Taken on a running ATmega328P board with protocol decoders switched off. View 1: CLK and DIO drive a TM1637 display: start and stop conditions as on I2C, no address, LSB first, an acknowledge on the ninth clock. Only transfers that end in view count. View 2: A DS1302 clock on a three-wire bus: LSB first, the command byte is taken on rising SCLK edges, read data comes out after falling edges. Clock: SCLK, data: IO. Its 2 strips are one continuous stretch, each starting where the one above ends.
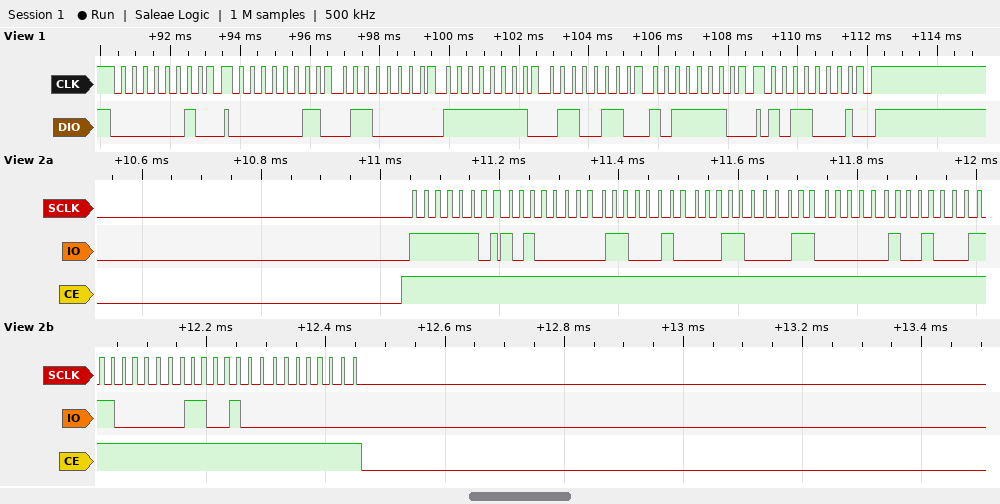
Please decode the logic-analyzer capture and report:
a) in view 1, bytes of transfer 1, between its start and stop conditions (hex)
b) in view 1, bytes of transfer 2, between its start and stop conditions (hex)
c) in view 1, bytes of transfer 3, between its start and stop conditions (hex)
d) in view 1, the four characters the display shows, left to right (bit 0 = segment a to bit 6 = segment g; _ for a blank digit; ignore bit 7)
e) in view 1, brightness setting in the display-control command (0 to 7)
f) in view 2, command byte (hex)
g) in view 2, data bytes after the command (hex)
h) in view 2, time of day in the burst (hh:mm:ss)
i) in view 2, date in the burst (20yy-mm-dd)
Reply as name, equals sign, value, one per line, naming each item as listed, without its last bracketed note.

in view 1, bytes of transfer 1, between its start and stop conditions = 40
in view 1, bytes of transfer 2, between its start and stop conditions = C0 06 FF 66 7D
in view 1, bytes of transfer 3, between its start and stop conditions = 8D
in view 1, the four characters the display shows, left to right = 1846
in view 1, brightness setting in the display-control command = 5
in view 2, command byte = 0xBF
in view 2, data bytes after the command = 05 46 18 06 12 07 26 00
in view 2, time of day in the burst = 18:46:05
in view 2, date in the burst = 2026-12-06
